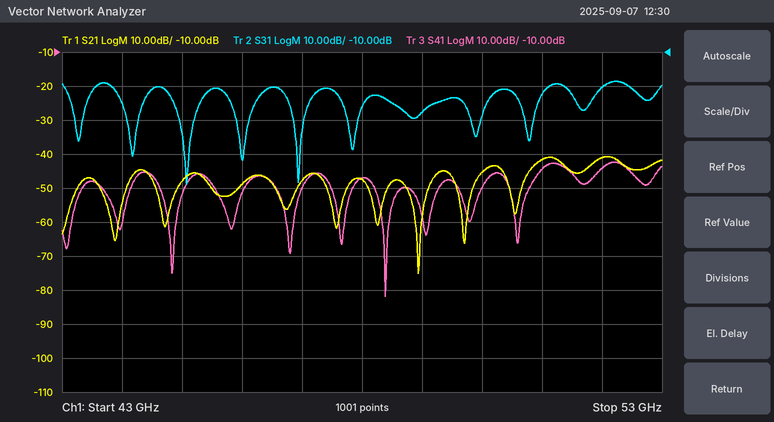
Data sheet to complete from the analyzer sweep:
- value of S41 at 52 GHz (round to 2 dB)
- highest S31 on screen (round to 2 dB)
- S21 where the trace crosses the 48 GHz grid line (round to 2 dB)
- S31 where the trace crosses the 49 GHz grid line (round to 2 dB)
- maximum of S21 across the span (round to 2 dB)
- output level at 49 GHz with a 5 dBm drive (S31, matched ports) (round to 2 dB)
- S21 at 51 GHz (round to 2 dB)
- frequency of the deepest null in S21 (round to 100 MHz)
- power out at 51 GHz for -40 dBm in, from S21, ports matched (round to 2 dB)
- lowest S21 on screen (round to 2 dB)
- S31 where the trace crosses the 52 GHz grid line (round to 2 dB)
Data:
-44 dB
-18 dB
-48 dB
-28 dB
-40 dB
-22 dBm
-42 dB
48.9 GHz
-82 dBm
-76 dB
-20 dB
